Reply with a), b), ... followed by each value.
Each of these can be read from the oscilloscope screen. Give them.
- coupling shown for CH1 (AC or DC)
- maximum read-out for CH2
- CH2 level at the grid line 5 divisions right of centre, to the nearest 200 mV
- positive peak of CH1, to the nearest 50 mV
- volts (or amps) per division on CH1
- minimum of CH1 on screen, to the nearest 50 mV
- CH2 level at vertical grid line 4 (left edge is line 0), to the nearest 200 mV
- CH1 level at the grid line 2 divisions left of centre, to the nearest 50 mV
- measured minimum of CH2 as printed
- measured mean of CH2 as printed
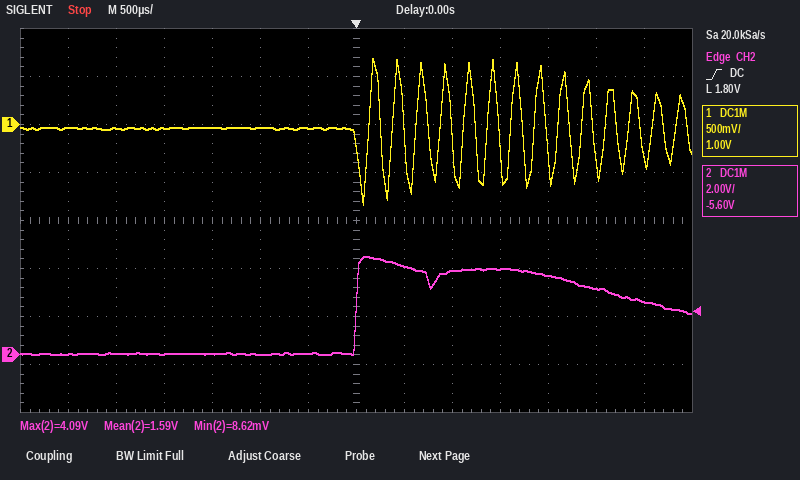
a) DC
b) 4.09 V
c) 2.8 V
d) 700 mV
e) 500 mV
f) -850 mV
g) 0.0 V
h) -50 mV
i) 8.62 mV
j) 1.59 V
